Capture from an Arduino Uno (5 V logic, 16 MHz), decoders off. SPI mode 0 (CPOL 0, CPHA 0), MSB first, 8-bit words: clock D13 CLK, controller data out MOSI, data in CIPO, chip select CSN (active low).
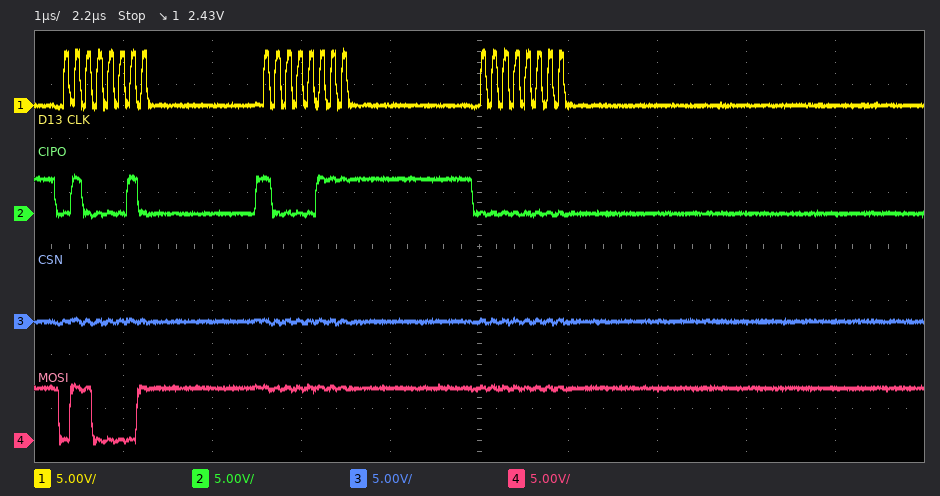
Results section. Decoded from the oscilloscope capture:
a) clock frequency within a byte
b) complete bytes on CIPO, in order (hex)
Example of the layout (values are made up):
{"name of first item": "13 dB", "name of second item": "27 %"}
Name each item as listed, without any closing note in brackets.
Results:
{"clock frequency within a byte": "8 MHz", "complete bytes on CIPO, in order": "42 87 00"}
